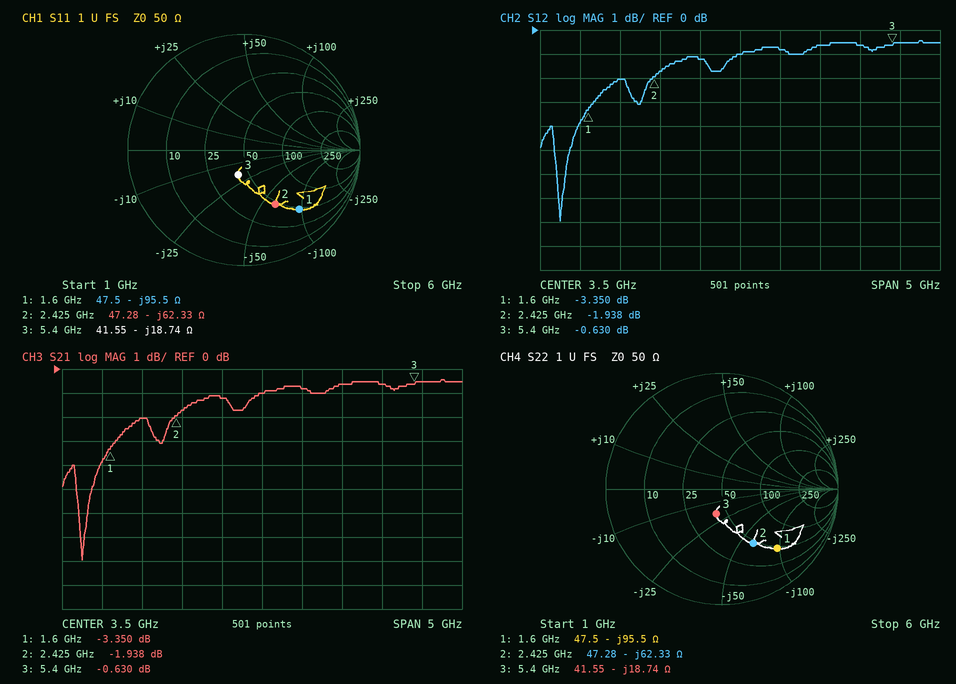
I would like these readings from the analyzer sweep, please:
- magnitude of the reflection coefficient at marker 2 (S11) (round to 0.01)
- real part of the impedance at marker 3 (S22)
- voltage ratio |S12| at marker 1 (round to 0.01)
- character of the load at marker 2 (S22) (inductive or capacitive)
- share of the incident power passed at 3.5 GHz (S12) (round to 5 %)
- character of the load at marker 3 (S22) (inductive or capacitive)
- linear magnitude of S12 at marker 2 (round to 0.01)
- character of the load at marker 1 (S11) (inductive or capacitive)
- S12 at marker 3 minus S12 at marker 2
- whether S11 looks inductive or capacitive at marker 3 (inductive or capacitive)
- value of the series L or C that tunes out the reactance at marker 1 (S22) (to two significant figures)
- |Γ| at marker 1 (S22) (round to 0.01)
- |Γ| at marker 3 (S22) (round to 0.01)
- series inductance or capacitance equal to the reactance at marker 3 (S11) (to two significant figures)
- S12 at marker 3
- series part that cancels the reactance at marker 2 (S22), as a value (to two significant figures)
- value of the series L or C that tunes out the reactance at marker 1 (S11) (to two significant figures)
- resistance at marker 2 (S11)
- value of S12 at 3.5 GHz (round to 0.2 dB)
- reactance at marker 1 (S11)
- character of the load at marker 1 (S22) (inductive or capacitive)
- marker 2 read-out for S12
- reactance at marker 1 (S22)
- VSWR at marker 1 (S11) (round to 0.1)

0.54
41.55 Ω
0.68
capacitive
80 %
capacitive
0.80
capacitive
1.308 dB
capacitive
9.5 nH
0.70
0.22
1.6 pF
-0.630 dB
4.1 nH
9.5 nH
47.28 Ω
-1.0 dB
-95.5 Ω
capacitive
-1.938 dB
-95.5 Ω
5.7
